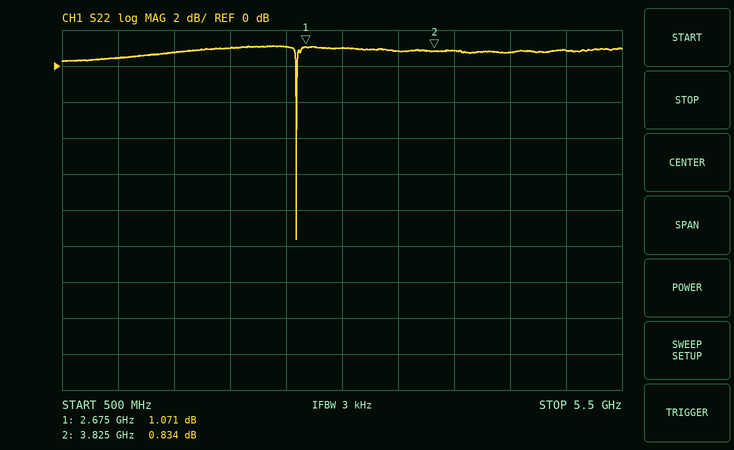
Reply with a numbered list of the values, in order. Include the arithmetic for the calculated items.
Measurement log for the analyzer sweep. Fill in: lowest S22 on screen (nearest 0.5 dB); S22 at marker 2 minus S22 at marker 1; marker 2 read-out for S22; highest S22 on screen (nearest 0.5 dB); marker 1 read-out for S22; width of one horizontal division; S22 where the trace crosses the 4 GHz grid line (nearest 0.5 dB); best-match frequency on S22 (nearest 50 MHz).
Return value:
1. -9.5 dB
2. 0.834 − (1.071) = -0.237 dB
3. 0.834 dB
4. 1.0 dB
5. 1.071 dB
6. 500 MHz
7. 1.0 dB
8. 2.60 GHz
